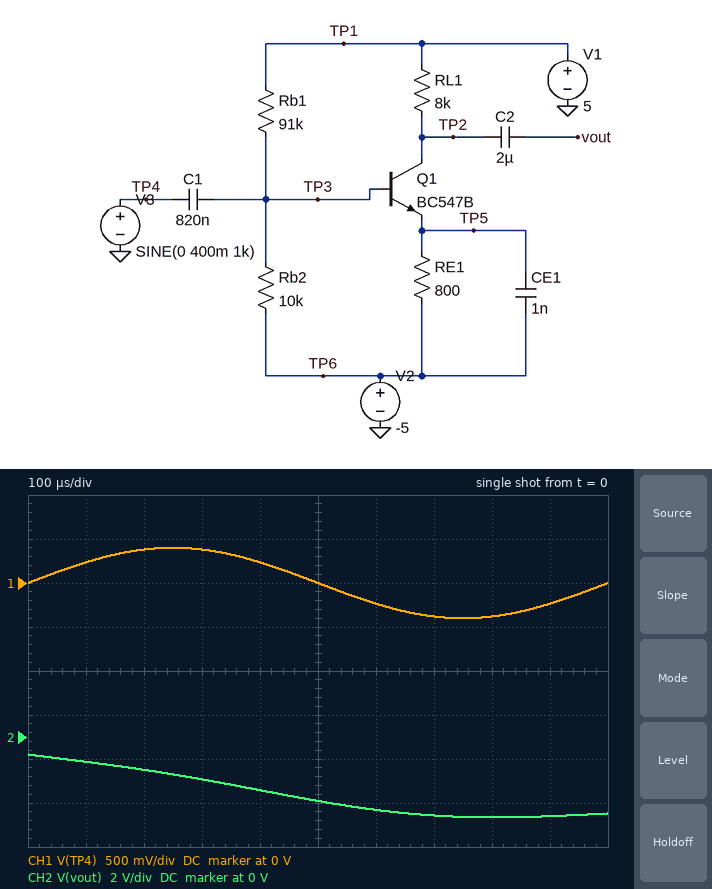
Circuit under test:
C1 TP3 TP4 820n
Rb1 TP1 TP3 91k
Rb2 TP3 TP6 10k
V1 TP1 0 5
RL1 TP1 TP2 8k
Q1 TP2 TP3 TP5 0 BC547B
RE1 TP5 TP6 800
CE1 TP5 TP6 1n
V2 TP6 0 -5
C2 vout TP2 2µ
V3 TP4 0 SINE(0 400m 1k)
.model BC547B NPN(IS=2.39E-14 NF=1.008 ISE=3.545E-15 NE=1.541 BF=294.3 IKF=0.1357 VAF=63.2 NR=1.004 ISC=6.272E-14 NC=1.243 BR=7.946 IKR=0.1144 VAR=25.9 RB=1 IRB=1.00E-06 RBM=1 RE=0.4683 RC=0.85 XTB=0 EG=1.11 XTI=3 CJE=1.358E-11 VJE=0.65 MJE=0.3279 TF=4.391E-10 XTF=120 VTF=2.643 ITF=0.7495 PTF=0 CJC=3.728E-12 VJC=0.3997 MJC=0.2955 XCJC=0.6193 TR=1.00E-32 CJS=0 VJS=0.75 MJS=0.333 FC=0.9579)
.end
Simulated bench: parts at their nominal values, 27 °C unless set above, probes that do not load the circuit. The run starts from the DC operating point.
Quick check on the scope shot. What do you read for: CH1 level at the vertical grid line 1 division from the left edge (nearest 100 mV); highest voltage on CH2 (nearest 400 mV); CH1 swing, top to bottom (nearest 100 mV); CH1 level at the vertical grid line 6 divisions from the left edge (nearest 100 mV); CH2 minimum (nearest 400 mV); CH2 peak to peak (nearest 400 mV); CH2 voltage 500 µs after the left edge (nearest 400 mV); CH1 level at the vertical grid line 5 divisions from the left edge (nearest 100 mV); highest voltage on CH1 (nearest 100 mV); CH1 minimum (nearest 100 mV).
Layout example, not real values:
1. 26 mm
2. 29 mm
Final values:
1. 200 mV
2. -800 mV
3. 800 mV
4. -200 mV
5. -3.6 V
6. 2.8 V
7. -2.8 V
8. 0 V
9. 400 mV
10. -400 mV
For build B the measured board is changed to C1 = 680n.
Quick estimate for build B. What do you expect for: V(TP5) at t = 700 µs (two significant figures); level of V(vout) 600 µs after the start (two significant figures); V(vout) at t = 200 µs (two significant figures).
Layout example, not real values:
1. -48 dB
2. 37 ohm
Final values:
1. -3.8 V
2. -3.5 V
3. -1.7 V
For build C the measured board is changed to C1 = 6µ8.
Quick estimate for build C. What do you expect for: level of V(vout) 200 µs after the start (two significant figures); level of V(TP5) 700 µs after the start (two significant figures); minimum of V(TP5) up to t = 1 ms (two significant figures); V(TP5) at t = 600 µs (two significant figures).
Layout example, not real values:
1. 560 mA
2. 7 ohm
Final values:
1. -510 mV
2. -1.6 V
3. -1.7 V
4. -1.4 V
